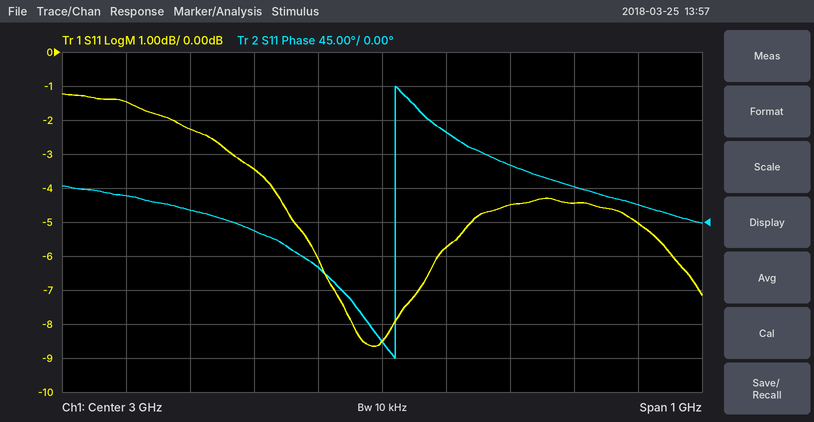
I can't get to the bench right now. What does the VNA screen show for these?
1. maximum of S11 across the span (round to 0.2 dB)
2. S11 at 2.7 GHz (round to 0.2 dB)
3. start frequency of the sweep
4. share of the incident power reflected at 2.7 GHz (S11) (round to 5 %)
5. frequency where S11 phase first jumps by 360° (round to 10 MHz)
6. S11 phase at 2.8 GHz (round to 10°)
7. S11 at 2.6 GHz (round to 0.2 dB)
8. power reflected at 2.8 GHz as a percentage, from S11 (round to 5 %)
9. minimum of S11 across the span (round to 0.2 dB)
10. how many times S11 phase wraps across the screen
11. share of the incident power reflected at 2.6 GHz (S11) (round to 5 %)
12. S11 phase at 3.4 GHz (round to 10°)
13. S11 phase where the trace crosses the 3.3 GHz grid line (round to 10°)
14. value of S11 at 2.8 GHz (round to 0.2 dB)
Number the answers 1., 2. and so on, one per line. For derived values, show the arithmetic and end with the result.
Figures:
1. -1.2 dB
2. -2.2 dB
3. 2.5 GHz
4. 10^(-2.2/10) ≈ 60 %
5. 3.02 GHz
6. -10°
7. -1.4 dB
8. 10^(-3.4/10) ≈ 45.7 %, so 45 % to the nearest 5 %
9. -8.6 dB
10. 1
11. 10^(-1.4/10) ≈ 72.4 %, so 70 % to the nearest 5 %
12. 20°
13. 50°
14. -3.4 dB
